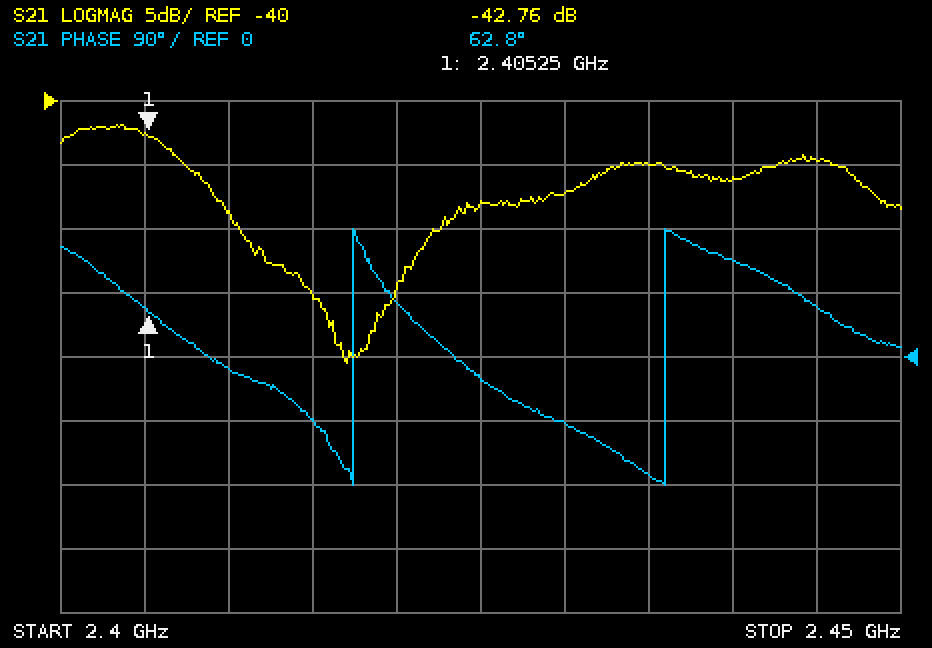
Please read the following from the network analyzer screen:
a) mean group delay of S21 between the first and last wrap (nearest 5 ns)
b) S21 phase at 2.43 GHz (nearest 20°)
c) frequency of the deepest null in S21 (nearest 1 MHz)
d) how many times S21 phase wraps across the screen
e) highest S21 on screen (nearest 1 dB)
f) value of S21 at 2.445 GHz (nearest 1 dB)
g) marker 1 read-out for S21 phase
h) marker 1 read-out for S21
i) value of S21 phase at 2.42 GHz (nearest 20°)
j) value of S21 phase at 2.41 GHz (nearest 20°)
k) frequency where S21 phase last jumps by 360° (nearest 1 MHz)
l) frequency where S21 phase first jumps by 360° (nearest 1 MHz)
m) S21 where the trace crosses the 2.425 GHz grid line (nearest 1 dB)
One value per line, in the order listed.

55 ns
-100°
2.417 GHz
2
-42 dB
-45 dB
62.8°
-42.76 dB
80°
-20°
2.436 GHz
2.417 GHz
-48 dB
